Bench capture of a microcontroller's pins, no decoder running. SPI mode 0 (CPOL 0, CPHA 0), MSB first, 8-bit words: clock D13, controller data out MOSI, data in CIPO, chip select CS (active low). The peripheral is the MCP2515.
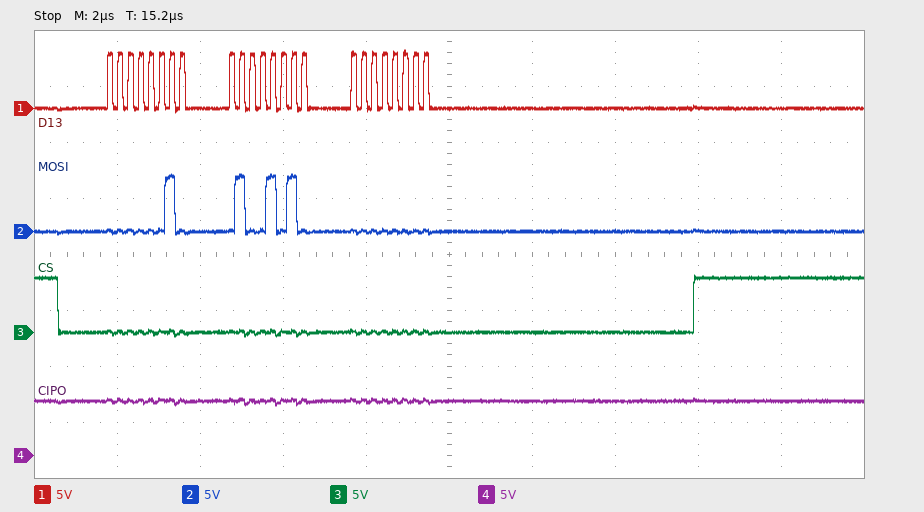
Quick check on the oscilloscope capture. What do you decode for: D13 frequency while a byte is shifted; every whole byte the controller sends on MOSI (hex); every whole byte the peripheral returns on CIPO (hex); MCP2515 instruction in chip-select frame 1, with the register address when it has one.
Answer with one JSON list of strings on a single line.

["4 MHz", "02 4A 00", "FF FF FF", "WRITE 0x4A"]
